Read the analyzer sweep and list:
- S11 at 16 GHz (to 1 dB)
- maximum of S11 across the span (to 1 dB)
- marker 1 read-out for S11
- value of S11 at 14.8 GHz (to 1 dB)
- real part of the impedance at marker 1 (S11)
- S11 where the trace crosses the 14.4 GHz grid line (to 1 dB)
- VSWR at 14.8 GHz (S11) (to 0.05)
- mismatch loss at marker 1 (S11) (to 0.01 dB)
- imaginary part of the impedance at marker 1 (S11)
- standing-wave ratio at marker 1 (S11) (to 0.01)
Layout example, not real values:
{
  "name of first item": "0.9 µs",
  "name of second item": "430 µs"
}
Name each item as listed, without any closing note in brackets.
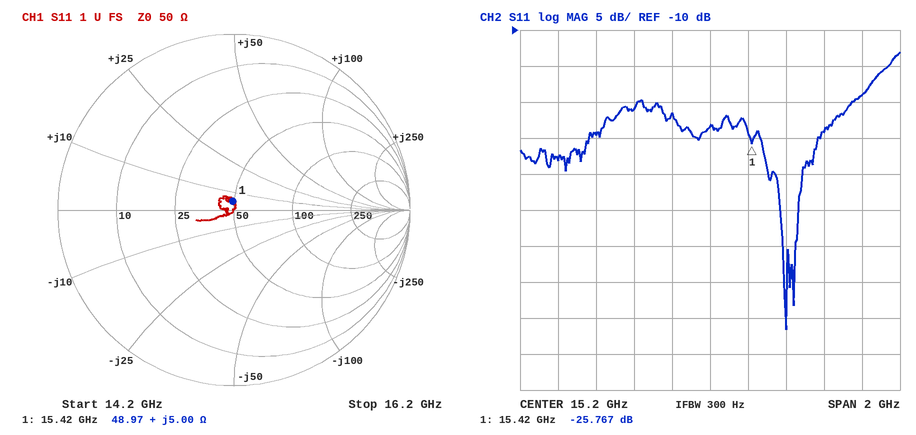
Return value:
{
  "S11 at 16 GHz": "-19 dB",
  "maximum of S11 across the span": "-13 dB",
  "marker 1 read-out for S11": "-25.767 dB",
  "value of S11 at 14.8 GHz": "-21 dB",
  "real part of the impedance at marker 1": "48.97 Ω",
  "S11 where the trace crosses the 14.4 GHz grid line": "-28 dB",
  "VSWR at 14.8 GHz (S11)": "1.20",
  "mismatch loss at marker 1 (S11)": "0.01 dB",
  "imaginary part of the impedance at marker 1": "+5.00 Ω",
  "standing-wave ratio at marker 1 (S11)": "1.11"
}
